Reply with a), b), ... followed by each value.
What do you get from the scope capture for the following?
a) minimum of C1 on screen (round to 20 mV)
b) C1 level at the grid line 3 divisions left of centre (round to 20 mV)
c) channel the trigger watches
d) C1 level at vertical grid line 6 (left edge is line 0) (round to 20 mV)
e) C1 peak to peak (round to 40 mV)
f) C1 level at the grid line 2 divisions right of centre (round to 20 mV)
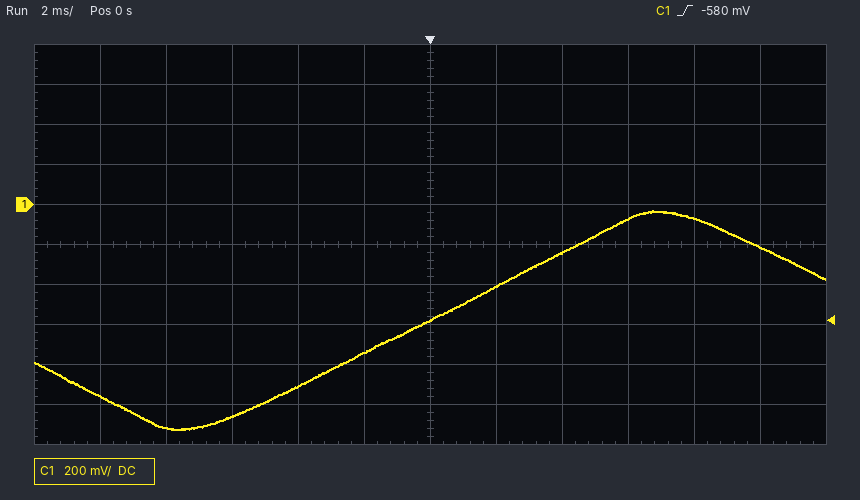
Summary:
a) -1.12 V
b) -1.06 V
c) C1
d) -580 mV
e) 1.08 V
f) -240 mV
